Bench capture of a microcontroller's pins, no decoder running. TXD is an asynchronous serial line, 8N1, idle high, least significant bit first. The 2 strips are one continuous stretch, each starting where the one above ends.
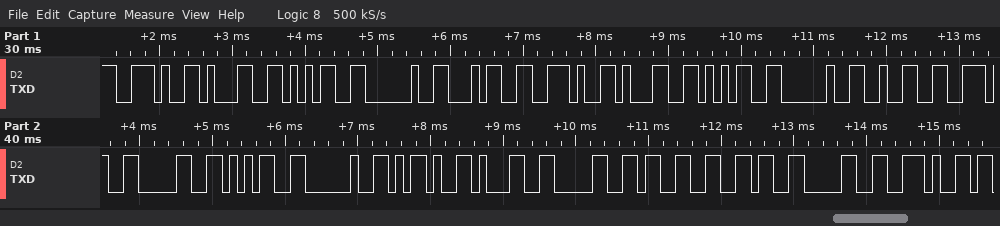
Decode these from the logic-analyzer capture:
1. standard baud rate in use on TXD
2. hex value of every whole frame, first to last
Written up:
9600 baud
0x2E 0x31 0x35 0x20 0x34 0x2E 0x31 0x35 0x20 0x32 0x2E 0x30 0x35 0x20 0x2D 0x31 0x30 0x33 0x36 0x30 0x2E
